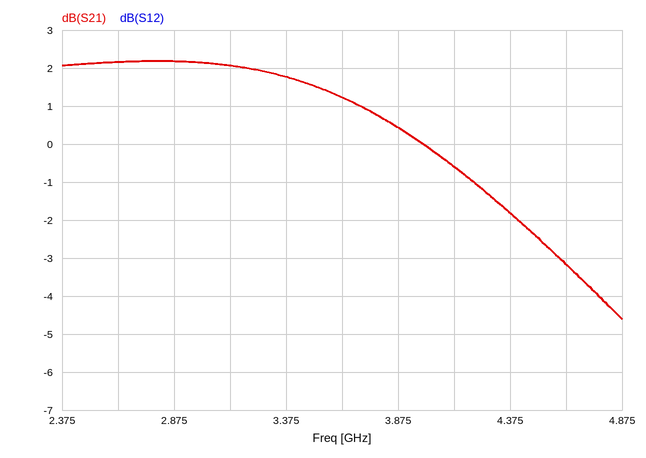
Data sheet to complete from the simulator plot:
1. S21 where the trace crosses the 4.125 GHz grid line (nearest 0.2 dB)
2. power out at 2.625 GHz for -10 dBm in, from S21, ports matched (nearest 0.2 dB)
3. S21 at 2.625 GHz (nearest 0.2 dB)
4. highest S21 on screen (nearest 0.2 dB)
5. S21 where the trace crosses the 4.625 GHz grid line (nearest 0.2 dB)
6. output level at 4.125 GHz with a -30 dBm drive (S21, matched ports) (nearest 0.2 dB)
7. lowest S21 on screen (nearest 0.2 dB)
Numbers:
-0.6 dB
-7.8 dBm
2.2 dB
2.2 dB
-3.2 dB
-30.6 dBm
-4.6 dB
